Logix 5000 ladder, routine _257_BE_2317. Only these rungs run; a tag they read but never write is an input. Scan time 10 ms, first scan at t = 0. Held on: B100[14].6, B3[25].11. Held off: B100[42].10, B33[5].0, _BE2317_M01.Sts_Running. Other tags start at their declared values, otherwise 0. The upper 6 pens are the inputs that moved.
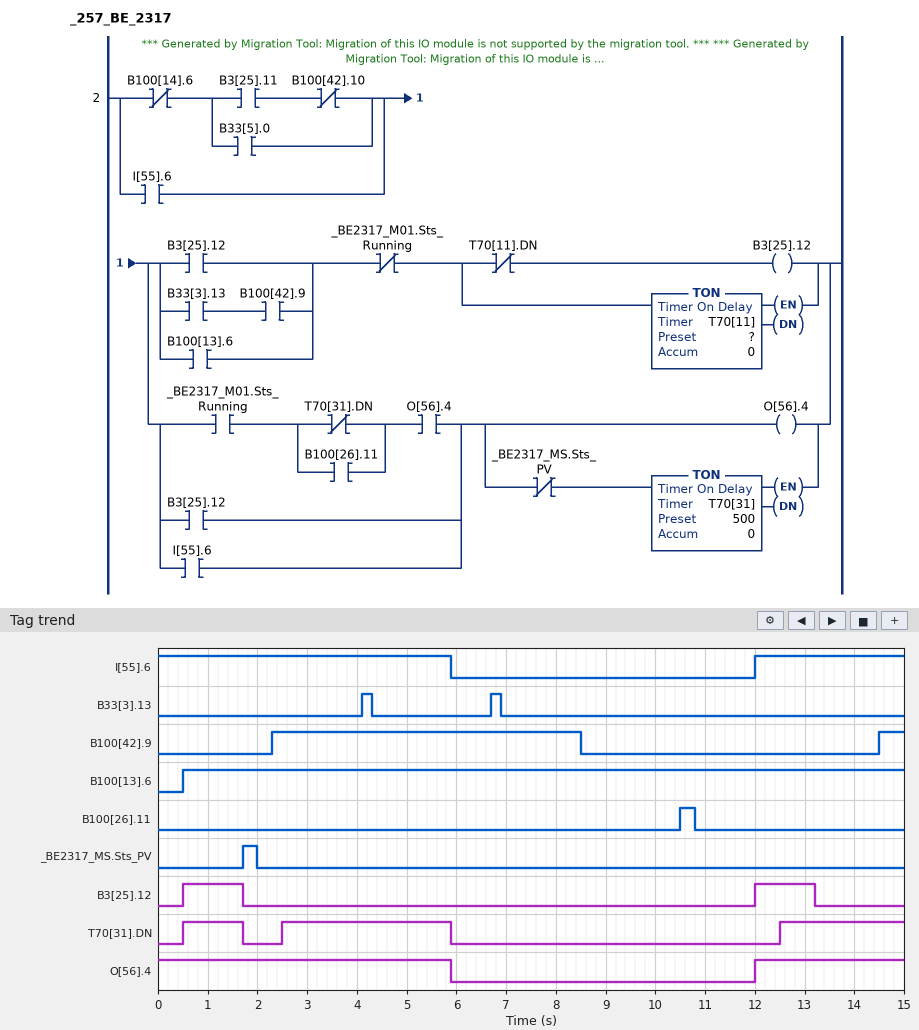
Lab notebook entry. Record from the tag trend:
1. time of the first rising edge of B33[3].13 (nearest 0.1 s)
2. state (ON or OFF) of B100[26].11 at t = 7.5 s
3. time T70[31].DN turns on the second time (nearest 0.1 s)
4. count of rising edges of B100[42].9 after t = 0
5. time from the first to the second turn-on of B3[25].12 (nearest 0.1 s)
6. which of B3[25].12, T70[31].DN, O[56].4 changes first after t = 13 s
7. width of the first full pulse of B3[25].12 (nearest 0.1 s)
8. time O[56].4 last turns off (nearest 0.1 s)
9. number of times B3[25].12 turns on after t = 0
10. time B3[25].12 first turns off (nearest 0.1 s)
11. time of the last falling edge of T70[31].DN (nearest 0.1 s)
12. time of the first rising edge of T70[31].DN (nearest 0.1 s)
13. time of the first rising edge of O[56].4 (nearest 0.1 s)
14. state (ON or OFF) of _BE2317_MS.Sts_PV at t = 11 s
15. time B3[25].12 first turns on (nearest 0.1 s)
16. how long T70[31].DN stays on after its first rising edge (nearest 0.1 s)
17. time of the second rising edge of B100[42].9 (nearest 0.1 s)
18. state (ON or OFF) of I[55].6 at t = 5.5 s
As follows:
4.1 s
OFF
2.5 s
2
11.5 s
B3[25].12
1.2 s
5.9 s
2
1.7 s
5.9 s
0.5 s
12.0 s
OFF
0.5 s
1.2 s
14.5 s
ON
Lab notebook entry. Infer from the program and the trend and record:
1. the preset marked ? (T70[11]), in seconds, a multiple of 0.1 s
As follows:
1.2 s
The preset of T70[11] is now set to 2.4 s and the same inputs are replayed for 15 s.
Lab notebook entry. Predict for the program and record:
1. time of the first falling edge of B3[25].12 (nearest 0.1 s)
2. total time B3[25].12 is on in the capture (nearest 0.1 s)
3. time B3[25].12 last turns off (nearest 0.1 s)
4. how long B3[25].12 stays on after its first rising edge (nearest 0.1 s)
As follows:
2.9 s
4.8 s
14.4 s
2.4 s
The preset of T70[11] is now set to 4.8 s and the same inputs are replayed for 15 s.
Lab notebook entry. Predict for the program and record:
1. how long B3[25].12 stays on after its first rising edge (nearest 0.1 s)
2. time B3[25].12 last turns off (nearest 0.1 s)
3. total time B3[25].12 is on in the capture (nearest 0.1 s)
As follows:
4.8 s
5.3 s
7.8 s
